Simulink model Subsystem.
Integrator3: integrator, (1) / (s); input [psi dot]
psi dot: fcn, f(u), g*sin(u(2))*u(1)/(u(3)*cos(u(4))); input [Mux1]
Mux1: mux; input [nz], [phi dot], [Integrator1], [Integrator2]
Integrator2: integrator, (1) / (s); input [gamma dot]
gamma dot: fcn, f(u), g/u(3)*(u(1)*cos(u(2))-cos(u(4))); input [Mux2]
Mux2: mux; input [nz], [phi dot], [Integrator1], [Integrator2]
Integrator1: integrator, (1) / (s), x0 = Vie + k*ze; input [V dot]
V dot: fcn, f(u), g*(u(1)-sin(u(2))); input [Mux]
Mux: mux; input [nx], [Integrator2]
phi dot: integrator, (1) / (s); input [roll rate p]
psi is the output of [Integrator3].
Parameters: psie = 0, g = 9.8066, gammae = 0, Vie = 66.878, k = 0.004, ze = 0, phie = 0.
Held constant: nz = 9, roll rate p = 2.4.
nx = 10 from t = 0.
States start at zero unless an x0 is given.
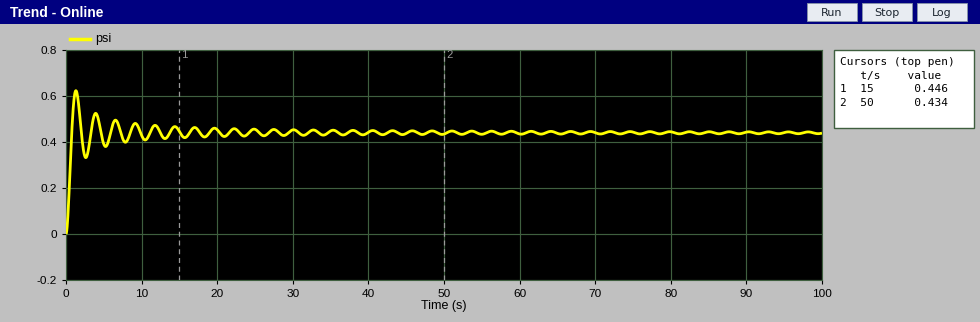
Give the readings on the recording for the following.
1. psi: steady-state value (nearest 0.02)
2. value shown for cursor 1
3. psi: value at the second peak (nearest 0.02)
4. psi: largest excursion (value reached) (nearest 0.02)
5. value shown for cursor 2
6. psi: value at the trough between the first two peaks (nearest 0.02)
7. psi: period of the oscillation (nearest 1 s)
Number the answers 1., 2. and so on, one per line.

1. 0.44
2. 0.446
3. 0.52
4. 0.62
5. 0.434
6. 0.34
7. 3 s
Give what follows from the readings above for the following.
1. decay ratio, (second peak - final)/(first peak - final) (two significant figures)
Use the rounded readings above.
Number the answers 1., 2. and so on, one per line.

1. 0.44
